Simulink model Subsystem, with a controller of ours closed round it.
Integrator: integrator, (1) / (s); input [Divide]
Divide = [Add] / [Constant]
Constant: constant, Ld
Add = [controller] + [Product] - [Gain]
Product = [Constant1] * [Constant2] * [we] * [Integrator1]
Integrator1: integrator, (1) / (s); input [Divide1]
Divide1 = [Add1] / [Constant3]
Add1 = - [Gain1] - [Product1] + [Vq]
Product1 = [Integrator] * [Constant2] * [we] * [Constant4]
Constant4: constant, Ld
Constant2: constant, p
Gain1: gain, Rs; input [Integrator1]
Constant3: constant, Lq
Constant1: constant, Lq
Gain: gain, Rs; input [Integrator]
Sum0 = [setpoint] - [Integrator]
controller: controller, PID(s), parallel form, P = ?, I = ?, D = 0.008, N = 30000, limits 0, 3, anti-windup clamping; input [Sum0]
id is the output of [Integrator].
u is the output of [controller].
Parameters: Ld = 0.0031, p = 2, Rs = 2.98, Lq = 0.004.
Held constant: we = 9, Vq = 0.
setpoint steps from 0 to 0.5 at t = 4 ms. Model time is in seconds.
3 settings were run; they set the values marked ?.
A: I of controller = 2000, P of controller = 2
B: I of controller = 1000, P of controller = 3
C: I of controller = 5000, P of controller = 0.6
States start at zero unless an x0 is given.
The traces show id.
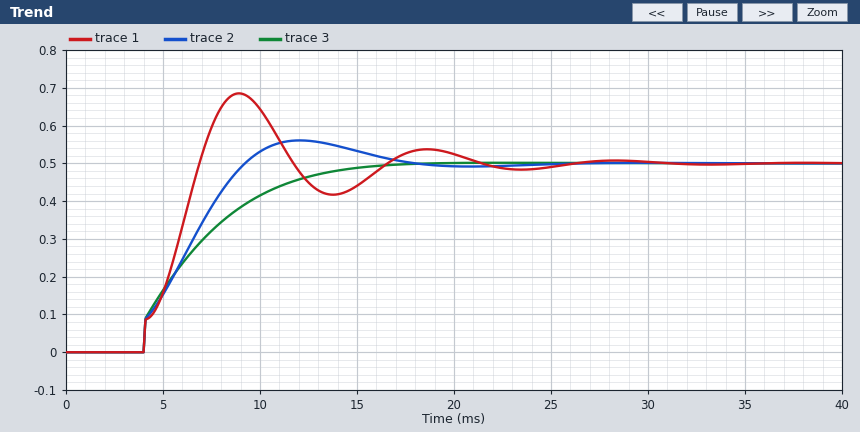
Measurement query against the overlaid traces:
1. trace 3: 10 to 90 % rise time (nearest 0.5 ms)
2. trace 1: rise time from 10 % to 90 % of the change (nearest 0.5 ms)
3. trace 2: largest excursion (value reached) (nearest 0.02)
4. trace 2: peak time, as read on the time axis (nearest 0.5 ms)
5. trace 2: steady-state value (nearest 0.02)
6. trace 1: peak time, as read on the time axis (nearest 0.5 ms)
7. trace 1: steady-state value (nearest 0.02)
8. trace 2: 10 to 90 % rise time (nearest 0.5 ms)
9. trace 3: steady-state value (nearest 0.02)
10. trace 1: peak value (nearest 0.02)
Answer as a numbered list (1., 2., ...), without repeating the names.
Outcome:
1. 7.5 ms
2. 2.5 ms
3. 0.56
4. 12.0 ms
5. 0.50
6. 9.0 ms
7. 0.50
8. 4.5 ms
9. 0.50
10. 0.68
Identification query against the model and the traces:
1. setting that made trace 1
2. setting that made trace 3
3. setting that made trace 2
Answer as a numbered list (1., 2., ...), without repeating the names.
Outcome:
1. C
2. B
3. A
